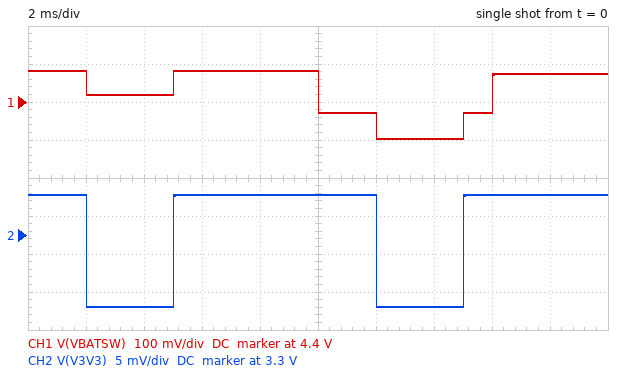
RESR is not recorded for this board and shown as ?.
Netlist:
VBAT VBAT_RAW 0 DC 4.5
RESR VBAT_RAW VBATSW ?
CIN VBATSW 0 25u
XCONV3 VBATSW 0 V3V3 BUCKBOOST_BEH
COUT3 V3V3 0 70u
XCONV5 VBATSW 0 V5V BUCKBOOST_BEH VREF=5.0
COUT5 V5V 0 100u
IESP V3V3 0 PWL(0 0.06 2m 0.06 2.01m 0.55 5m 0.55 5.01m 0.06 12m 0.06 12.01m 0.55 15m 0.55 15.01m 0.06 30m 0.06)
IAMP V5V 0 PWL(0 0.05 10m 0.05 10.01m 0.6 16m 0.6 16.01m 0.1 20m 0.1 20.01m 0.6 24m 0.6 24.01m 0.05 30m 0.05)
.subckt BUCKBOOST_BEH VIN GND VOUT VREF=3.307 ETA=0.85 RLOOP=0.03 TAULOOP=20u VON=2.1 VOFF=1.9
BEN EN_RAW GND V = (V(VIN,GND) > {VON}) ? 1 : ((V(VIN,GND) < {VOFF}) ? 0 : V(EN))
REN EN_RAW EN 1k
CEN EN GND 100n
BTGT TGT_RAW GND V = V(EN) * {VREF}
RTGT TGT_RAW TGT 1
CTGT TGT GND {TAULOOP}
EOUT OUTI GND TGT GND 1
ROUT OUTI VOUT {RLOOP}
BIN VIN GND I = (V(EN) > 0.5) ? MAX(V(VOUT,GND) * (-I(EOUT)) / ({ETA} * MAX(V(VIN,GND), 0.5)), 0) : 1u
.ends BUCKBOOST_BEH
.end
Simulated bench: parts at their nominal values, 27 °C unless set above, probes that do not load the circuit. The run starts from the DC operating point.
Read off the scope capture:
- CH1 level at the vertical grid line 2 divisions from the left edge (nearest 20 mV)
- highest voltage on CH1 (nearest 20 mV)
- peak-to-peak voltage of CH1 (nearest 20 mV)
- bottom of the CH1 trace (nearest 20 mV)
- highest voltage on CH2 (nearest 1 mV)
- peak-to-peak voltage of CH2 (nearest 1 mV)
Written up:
4.42 V
4.48 V
180 mV
4.30 V
3.305 V
15 mV
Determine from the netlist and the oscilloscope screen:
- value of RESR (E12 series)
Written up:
0.15 Ω
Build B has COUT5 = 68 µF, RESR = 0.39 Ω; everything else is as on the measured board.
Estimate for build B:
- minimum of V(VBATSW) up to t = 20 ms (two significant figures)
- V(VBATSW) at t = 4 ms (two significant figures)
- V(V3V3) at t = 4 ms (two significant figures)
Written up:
3.9 V
4.3 V
3.3 V
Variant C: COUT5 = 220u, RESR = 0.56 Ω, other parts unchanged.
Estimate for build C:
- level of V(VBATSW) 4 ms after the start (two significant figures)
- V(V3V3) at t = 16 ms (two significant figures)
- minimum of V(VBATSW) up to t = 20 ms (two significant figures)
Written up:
4.2 V
3.3 V
3.6 V
